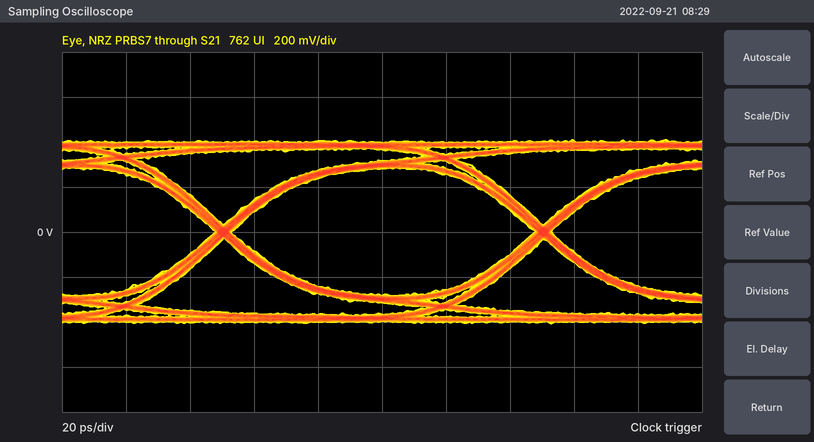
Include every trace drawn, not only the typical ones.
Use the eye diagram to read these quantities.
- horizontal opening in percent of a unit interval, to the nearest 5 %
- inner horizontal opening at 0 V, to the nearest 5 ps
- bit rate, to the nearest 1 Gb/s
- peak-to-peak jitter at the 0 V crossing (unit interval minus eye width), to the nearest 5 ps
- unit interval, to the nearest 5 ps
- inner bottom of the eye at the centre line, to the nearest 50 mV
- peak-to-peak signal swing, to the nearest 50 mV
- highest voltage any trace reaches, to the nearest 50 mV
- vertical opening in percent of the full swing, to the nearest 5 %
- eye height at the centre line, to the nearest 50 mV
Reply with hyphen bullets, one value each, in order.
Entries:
- 95 %
- 95 ps
- 10 Gb/s
- 5 ps
- 100 ps
- -300 mV
- 800 mV
- 400 mV
- 70 %
- 550 mV
